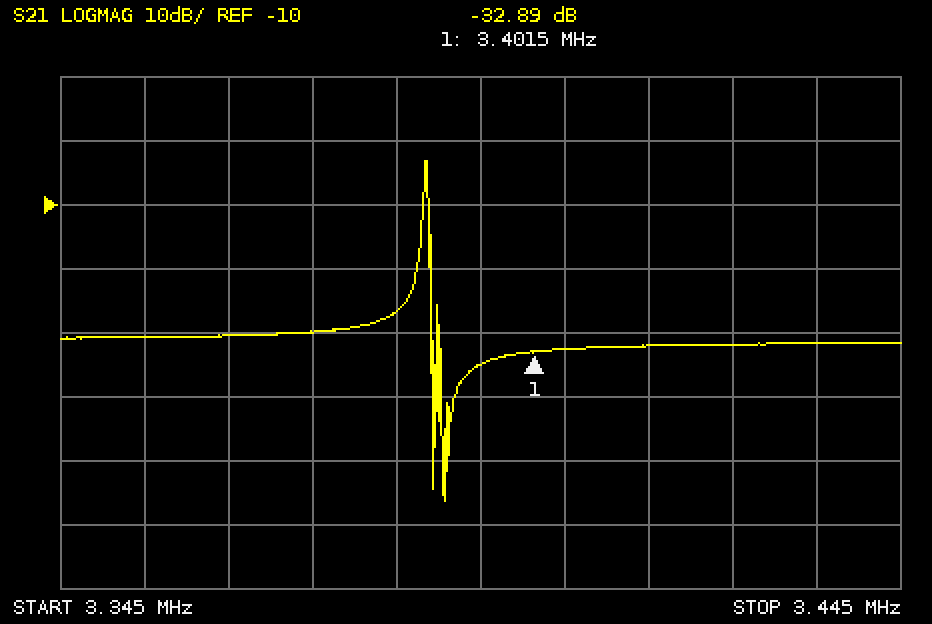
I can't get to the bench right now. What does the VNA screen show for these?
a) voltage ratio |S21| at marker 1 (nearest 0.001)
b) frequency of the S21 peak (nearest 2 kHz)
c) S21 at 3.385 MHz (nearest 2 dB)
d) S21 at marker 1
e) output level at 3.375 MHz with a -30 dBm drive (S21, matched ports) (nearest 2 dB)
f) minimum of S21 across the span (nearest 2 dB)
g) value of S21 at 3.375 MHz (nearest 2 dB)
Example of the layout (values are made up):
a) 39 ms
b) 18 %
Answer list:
a) 0.023
b) 3.388 MHz
c) -26 dB
d) -32.89 dB
e) -60 dBm
f) -56 dB
g) -30 dB
